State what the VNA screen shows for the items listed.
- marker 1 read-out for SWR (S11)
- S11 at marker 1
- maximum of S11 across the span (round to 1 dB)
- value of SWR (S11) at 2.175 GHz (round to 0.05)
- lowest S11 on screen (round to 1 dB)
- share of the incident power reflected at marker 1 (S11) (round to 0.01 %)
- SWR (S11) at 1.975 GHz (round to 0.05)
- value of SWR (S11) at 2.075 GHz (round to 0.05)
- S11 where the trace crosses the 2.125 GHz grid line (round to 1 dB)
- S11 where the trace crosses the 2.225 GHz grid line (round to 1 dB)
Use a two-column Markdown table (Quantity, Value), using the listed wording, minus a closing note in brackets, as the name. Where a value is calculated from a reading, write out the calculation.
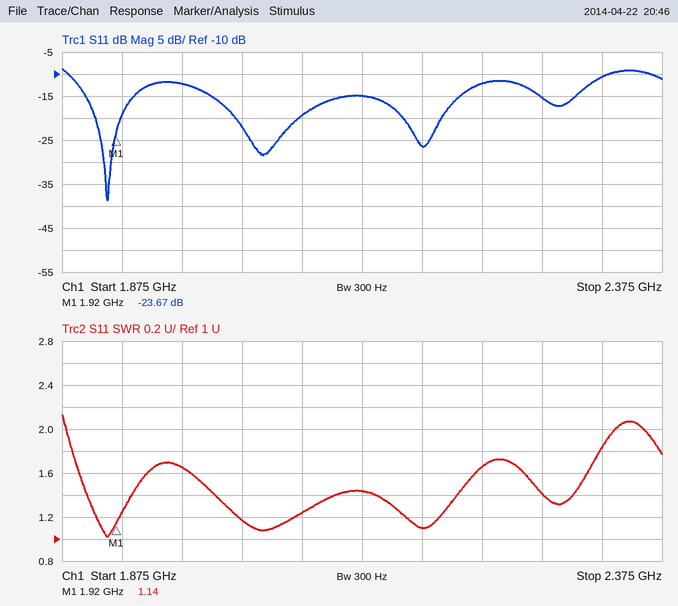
| Quantity | Value |
|---|---|
| marker 1 read-out for SWR | 1.14 |
| S11 at marker 1 | -23.67 dB |
| maximum of S11 across the span | -9 dB |
| value of SWR (S11) at 2.175 GHz | 1.10 |
| lowest S11 on screen | -39 dB |
| share of the incident power reflected at marker 1 (S11) | 10^(-23.67/10) ≈ 0.43 % |
| SWR (S11) at 1.975 GHz | 1.65 |
| value of SWR (S11) at 2.075 GHz | 1.25 |
| S11 where the trace crosses the 2.125 GHz grid line | -15 dB |
| S11 where the trace crosses the 2.225 GHz grid line | -12 dB |
